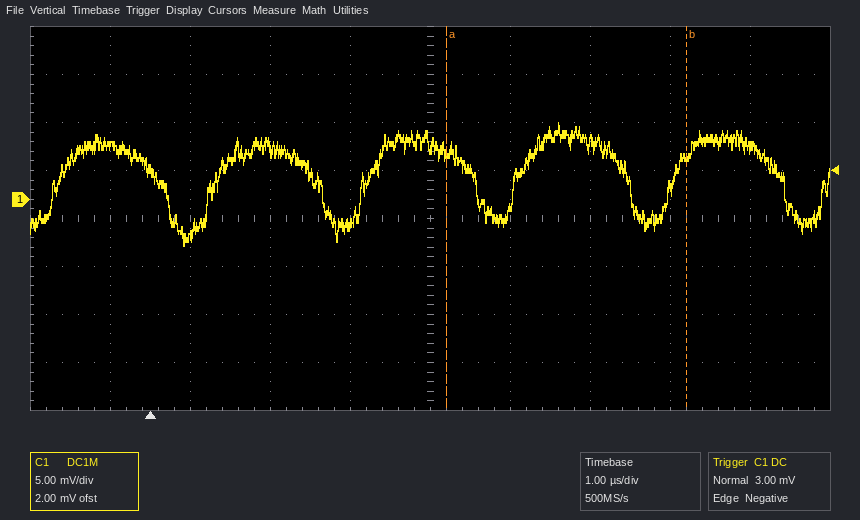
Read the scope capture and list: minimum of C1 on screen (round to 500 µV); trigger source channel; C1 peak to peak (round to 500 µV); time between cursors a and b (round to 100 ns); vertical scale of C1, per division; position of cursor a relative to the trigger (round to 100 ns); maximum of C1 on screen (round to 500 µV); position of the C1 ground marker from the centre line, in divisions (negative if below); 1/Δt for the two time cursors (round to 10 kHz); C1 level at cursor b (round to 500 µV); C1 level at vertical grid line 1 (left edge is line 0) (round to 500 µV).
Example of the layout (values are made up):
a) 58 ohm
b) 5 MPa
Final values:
a) -5.0 mV
b) C1
c) 13.0 mV
d) 3.0 µs
e) 5 mV
f) +3.7 µs
g) 8.0 mV
h) +0.4 div
i) 330 kHz
j) 4.5 mV
k) 5.5 mV
